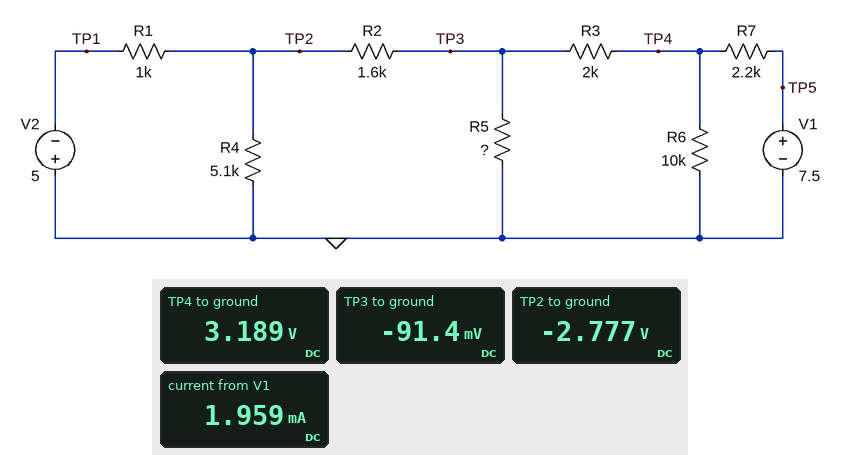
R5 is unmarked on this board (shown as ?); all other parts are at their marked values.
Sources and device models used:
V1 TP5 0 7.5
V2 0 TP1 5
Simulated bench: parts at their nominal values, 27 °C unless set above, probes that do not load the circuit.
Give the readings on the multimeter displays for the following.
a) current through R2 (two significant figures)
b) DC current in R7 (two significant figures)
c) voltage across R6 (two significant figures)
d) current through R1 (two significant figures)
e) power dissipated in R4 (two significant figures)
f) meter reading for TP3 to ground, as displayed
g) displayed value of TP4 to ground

1.7 mA
2.0 mA
3.2 V
2.2 mA
1.5 mW
-91.4 mV
3.189 V
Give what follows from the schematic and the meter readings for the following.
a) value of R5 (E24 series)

2.4 kΩ
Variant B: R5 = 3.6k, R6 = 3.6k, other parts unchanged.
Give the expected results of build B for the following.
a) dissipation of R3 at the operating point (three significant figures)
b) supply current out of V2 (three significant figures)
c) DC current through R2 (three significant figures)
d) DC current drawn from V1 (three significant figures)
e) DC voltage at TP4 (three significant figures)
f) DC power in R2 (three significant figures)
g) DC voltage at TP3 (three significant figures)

4.40 mW
2.14 mA
1.58 mA
2.21 mA
2.63 V
3.98 mW
-338 mV
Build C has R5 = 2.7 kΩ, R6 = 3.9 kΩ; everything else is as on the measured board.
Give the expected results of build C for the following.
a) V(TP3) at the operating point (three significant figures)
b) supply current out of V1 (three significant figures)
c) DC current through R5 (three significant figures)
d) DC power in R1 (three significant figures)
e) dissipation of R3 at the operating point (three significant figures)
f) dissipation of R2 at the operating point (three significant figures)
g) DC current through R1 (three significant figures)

-287 mV
2.18 mA
106 µA
4.65 mW
4.45 mW
4.09 mW
2.16 mA
